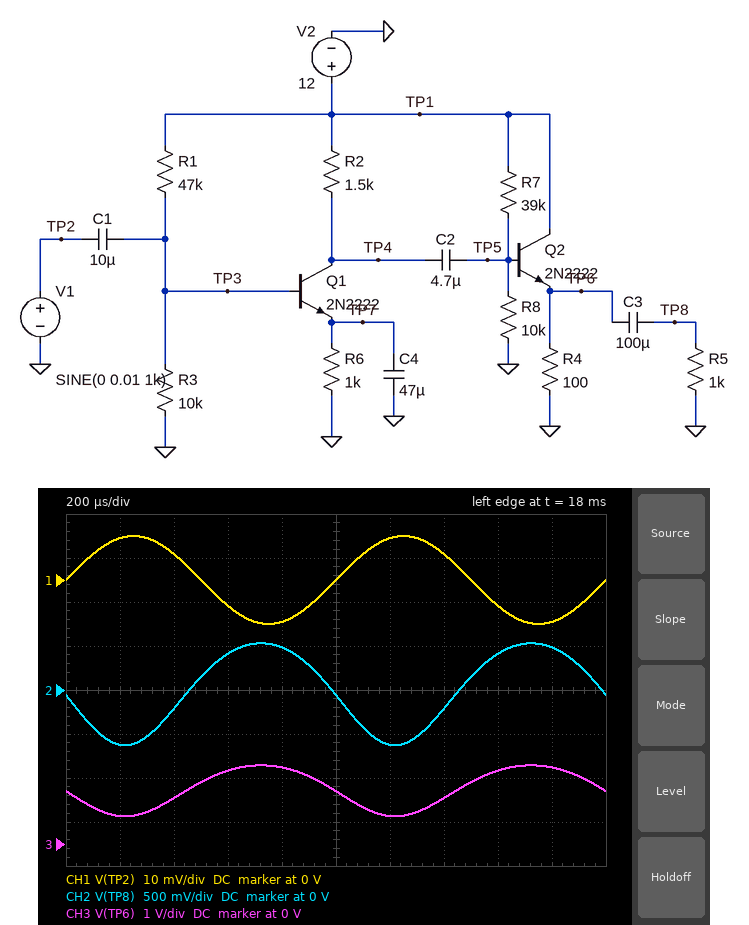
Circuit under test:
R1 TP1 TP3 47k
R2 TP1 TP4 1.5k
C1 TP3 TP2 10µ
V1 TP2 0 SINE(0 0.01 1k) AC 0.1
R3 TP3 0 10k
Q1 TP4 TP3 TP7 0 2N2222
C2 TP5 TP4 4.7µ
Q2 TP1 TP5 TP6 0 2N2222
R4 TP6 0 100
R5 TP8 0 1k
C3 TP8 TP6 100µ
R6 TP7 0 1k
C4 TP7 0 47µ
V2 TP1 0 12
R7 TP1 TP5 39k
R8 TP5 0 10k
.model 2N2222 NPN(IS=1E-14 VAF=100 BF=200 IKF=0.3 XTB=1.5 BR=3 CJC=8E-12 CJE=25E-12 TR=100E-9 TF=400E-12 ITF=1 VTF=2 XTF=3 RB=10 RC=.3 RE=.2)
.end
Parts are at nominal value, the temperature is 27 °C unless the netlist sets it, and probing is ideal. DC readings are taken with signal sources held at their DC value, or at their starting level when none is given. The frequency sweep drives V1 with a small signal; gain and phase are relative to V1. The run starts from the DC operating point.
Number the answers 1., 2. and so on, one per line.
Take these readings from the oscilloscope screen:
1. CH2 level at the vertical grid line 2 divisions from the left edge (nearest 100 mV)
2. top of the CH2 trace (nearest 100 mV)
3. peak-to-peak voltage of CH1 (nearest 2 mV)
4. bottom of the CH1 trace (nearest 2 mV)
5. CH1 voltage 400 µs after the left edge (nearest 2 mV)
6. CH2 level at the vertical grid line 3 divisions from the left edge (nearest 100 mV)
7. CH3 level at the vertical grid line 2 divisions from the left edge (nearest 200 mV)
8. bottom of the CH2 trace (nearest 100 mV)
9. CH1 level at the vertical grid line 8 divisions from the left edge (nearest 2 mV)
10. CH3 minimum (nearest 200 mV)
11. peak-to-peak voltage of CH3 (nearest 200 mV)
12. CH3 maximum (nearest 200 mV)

1. -200 mV
2. 500 mV
3. 20 mV
4. -10 mV
5. 6 mV
6. 400 mV
7. 1.0 V
8. -600 mV
9. -6 mV
10. 600 mV
11. 1.2 V
12. 1.8 V
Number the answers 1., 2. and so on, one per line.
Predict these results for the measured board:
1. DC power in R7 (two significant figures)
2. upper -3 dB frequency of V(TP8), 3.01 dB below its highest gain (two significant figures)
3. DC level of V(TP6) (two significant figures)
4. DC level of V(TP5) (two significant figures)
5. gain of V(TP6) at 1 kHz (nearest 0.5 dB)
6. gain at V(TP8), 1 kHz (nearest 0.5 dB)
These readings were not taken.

1. 2.6 mW
2. 9.6 MHz
3. 1.3 V
4. 2.0 V
5. 35.5 dB
6. 35.5 dB
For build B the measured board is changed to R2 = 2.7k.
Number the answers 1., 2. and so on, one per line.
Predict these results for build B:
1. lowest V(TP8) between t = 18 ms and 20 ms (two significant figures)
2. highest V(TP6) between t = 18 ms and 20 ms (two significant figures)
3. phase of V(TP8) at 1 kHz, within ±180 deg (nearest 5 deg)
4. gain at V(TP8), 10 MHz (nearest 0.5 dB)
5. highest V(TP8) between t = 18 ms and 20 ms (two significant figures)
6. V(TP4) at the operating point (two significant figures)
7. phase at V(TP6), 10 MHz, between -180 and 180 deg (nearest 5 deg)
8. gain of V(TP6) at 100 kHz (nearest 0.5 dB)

1. -950 mV
2. 2.1 V
3. -170 deg
4. 33.5 dB
5. 810 mV
6. 8.3 V
7. 120 deg
8. 39.0 dB
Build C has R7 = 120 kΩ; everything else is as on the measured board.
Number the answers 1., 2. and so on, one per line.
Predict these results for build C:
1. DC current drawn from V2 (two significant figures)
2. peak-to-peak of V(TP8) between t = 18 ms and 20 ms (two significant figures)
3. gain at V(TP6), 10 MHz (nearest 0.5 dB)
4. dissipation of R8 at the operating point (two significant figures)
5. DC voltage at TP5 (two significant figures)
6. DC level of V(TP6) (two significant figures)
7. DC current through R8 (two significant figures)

1. 3.5 mA
2. 670 mV
3. 30.0 dB
4. 72 µW
5. 850 mV
6. 180 mV
7. 85 µA
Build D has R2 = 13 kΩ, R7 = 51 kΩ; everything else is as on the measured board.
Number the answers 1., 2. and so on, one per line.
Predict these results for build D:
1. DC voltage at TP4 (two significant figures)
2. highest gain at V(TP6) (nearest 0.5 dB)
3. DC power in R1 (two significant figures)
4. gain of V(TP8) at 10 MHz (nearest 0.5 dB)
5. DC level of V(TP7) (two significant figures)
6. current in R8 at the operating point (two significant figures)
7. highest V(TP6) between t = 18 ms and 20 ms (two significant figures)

1. 960 mV
2. 9.5 dB
3. 2.3 mW
4. -1.5 dB
5. 910 mV
6. 160 µA
7. 1.3 V
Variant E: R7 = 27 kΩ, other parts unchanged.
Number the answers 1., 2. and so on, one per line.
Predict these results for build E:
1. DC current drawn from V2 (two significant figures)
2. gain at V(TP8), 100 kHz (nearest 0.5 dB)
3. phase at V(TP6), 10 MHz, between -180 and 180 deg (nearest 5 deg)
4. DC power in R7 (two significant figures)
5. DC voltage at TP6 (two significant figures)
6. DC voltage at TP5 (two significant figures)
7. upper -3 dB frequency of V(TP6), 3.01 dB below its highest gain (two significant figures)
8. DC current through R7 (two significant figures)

1. 20 mA
2. 35.5 dB
3. 135 deg
4. 3.3 mW
5. 1.9 V
6. 2.6 V
7. 9.9 MHz
8. 350 µA
